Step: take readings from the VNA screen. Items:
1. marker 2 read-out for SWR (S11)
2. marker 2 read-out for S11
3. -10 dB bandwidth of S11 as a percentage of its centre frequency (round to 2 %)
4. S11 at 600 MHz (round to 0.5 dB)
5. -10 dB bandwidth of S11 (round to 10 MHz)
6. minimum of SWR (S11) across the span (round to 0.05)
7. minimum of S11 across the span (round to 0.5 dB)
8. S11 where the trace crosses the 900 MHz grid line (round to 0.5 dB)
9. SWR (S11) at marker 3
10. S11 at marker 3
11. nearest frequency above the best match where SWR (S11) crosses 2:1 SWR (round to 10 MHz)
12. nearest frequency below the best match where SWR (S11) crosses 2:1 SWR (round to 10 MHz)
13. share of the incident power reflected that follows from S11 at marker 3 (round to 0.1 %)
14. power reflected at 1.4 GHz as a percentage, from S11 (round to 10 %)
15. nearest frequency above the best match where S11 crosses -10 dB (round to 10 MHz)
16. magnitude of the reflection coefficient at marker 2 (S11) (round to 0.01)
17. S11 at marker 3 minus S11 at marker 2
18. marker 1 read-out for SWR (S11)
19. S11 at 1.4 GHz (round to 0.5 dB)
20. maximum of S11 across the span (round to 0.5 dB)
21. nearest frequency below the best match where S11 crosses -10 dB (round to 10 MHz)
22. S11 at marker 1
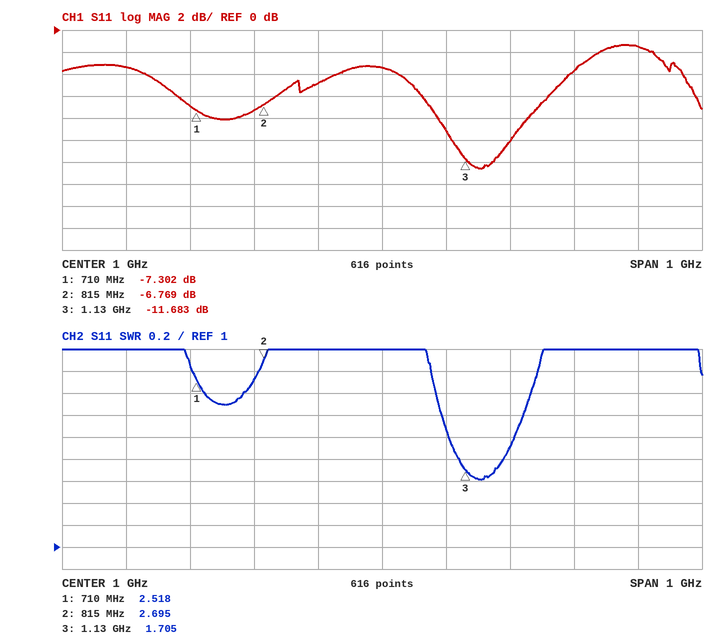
2.695
-6.769 dB
8 %
-3.5 dB
90 MHz
1.60
-12.5 dB
-5.0 dB
1.705
-11.683 dB
1.21 GHz
1.10 GHz
6.8 %
70 %
1.20 GHz
0.46
-4.914 dB
2.518
-1.5 dB
-1.5 dB
1.11 GHz
-7.302 dB
